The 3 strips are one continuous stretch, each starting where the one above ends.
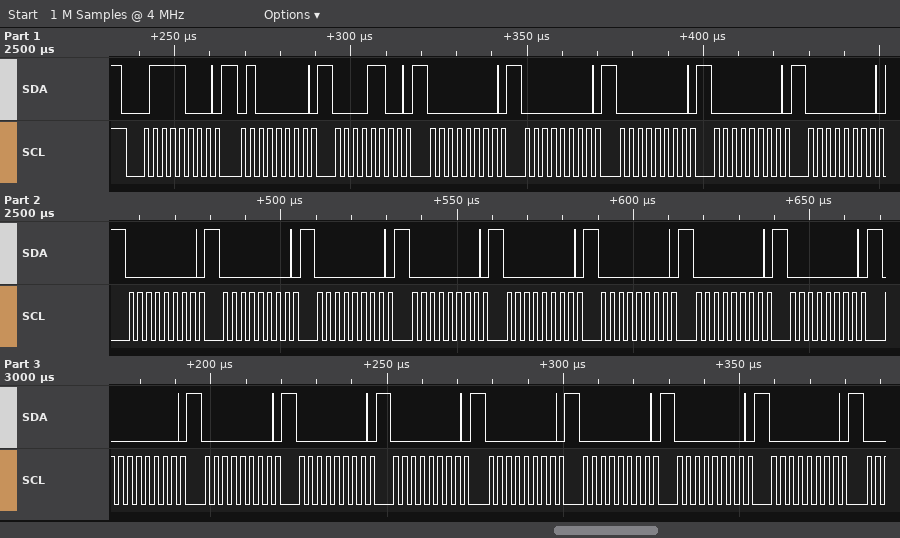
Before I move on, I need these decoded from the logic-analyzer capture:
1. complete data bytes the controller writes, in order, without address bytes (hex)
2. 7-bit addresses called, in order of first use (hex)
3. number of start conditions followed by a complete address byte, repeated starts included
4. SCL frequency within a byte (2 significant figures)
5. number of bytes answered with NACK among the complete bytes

40 0C 00 00 00 00 00 00 00 00 00 00 00 00 00 00 00 00 00 00 00 00 00
0x3C
1
400 kHz
0
